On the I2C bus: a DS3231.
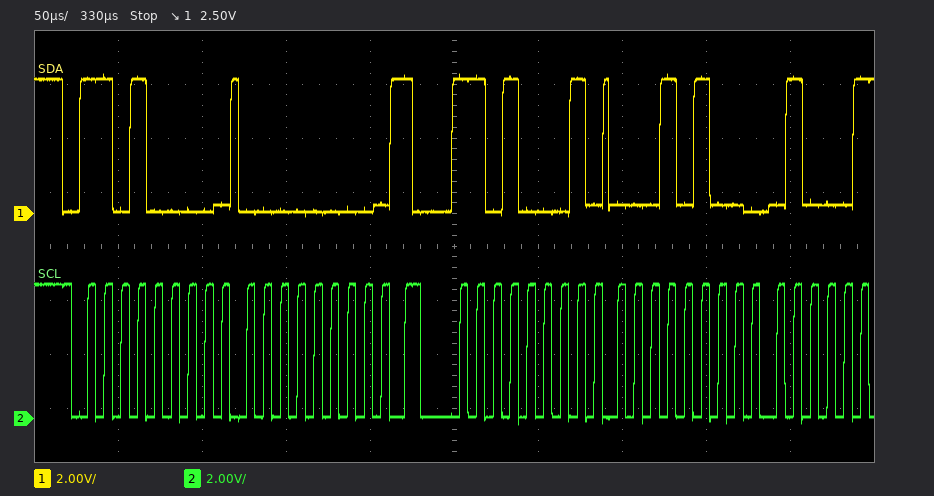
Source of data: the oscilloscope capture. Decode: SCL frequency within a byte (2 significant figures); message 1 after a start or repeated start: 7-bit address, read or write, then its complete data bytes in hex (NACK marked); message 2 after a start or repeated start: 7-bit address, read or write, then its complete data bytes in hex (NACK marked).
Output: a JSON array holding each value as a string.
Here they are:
["100 kHz", "0x68 write: 00", "0x68 read: 14"]
